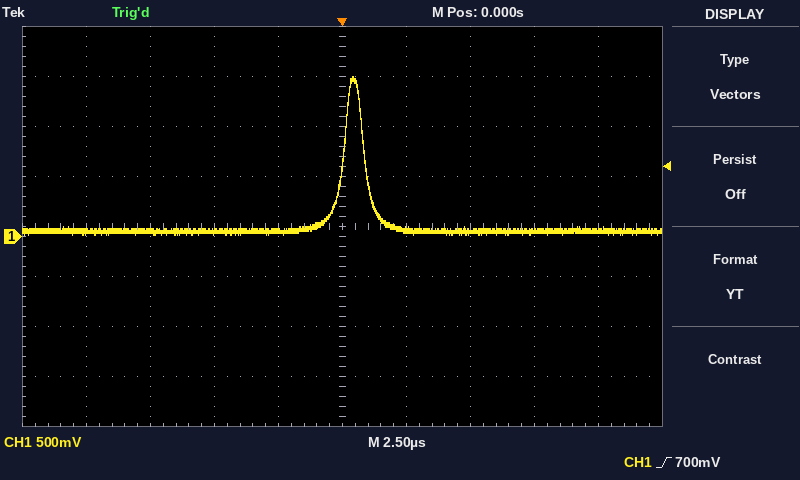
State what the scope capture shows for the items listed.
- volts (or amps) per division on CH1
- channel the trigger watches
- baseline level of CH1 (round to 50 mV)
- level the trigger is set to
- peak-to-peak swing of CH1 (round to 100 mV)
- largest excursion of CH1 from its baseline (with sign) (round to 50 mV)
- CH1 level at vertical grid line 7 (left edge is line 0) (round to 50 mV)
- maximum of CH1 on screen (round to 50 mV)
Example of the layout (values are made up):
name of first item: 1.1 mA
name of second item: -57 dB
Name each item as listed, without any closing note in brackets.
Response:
volts (or amps) per division on CH1: 500 mV
channel the trigger watches: CH1
baseline level of CH1: 50 mV
level the trigger is set to: 700 mV
peak-to-peak swing of CH1: 1.60 V
largest excursion of CH1 from its baseline (with sign): +1.55 V
CH1 level at vertical grid line 7 (left edge is line 0): 50 mV
maximum of CH1 on screen: 1.60 V
